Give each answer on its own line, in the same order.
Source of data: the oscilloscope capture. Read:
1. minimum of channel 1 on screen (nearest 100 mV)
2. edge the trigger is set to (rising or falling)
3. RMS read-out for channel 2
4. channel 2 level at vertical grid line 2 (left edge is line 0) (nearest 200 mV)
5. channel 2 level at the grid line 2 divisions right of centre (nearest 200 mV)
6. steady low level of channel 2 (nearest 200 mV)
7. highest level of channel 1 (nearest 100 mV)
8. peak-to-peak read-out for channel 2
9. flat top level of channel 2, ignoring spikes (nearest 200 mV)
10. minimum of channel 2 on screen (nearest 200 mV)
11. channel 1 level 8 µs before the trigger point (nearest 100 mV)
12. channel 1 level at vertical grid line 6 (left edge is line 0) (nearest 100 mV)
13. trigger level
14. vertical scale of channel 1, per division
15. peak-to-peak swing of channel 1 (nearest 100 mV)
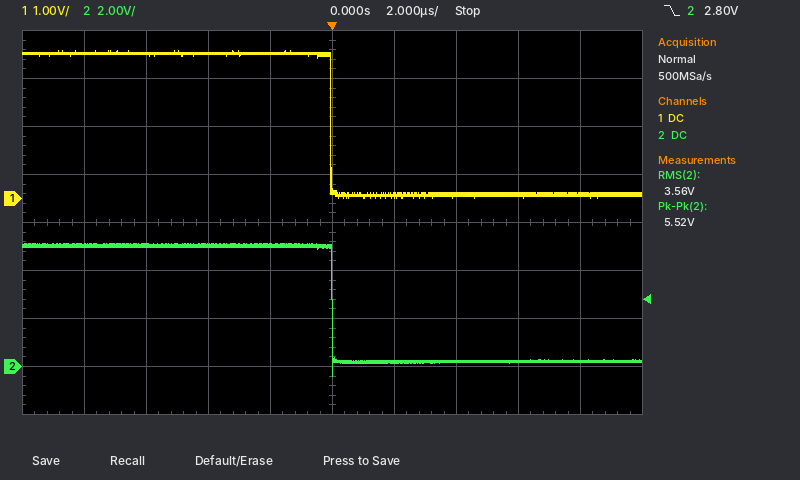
0.0 V
falling
3.56 V
5.0 V
200 mV
200 mV
3.1 V
5.52 V
5.0 V
-400 mV
3.0 V
100 mV
2.80 V
1 V
3.1 V
